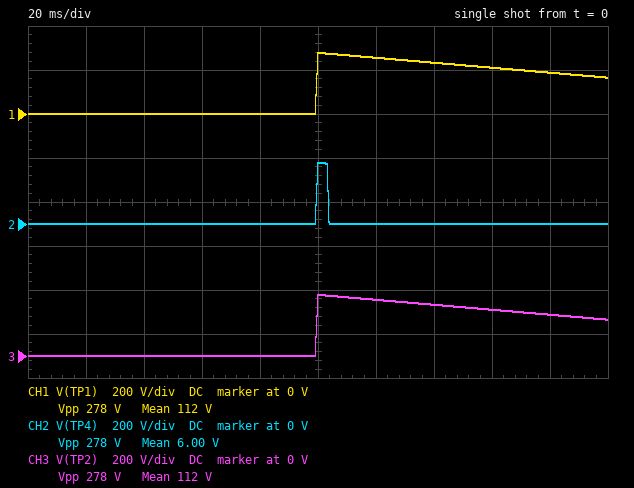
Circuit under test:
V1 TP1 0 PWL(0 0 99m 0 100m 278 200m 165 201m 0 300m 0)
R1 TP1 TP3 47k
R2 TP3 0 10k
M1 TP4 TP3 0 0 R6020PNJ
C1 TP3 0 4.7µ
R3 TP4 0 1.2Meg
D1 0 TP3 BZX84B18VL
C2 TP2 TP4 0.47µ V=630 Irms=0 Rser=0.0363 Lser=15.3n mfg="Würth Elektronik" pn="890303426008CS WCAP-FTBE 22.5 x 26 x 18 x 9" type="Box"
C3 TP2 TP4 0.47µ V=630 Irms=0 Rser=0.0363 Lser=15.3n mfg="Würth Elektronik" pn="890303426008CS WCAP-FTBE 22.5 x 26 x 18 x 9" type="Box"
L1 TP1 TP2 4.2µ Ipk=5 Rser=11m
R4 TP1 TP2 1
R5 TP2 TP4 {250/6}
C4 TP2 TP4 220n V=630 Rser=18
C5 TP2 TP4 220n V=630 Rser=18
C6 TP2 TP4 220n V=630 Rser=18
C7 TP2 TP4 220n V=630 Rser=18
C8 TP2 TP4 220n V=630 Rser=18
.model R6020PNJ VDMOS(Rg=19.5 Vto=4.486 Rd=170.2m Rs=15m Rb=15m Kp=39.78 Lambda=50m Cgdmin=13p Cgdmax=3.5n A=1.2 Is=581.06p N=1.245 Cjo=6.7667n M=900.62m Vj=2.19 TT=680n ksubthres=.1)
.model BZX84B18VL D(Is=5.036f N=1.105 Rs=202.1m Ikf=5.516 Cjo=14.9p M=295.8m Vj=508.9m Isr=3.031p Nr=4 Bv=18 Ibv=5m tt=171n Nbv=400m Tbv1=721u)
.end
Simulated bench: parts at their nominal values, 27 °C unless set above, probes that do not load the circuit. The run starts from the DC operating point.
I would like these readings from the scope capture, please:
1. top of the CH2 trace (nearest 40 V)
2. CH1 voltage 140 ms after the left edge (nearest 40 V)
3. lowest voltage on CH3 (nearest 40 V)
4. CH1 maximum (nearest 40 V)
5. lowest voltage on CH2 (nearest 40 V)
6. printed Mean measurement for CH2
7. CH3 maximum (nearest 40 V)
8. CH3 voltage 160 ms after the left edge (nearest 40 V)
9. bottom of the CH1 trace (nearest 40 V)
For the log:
280 V
240 V
0 V
280 V
0 V
6.00 V
280 V
200 V
0 V
